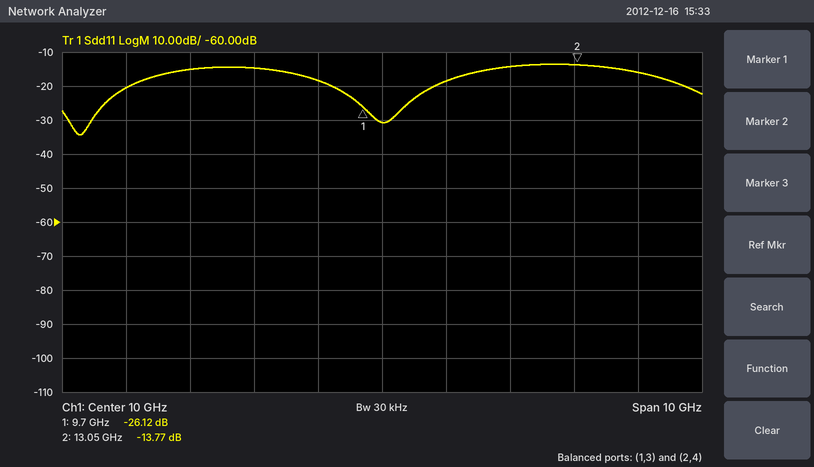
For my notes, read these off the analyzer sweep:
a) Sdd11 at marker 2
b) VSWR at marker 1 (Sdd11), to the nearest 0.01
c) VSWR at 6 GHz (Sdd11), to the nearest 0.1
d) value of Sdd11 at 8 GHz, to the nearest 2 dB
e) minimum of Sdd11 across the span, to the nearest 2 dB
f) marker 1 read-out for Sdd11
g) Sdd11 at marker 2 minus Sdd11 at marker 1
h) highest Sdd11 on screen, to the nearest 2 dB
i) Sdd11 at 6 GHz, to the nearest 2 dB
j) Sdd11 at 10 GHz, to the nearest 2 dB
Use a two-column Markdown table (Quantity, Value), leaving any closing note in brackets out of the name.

| Quantity | Value |
|---|---|
| Sdd11 at marker 2 | -13.77 dB |
| VSWR at marker 1 (Sdd11), to the nearest 0.01 | 1.10 |
| VSWR at 6 GHz (Sdd11), to the nearest 0.1 | 1.2 |
| value of Sdd11 at 8 GHz, to the nearest 2 dB | -14 dB |
| minimum of Sdd11 across the span, to the nearest 2 dB | -34 dB |
| marker 1 read-out for Sdd11 | -26.12 dB |
| Sdd11 at marker 2 minus Sdd11 at marker 1 | 12.35 dB |
| highest Sdd11 on screen, to the nearest 2 dB | -14 dB |
| Sdd11 at 6 GHz, to the nearest 2 dB | -20 dB |
| Sdd11 at 10 GHz, to the nearest 2 dB | -30 dB |
